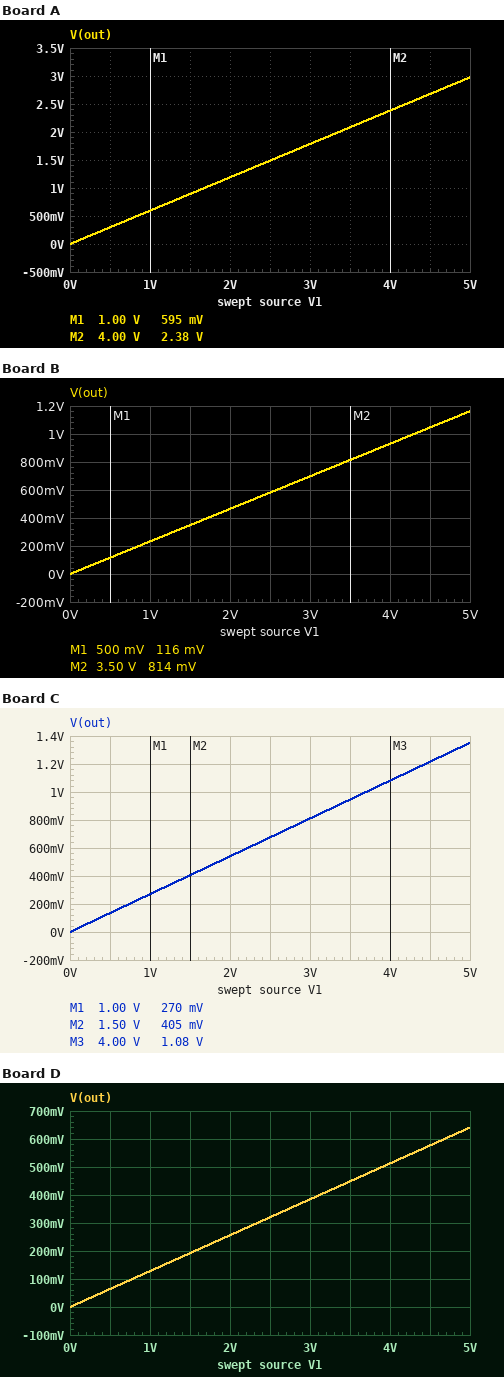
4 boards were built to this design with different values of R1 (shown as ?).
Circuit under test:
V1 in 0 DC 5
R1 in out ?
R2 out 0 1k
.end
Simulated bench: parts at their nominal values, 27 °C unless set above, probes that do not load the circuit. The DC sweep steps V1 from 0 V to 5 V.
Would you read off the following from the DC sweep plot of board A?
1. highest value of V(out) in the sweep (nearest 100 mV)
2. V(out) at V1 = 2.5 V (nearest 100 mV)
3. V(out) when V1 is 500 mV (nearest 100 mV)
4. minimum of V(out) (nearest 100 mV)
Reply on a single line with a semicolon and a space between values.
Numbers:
3.0 V; 1.5 V; 300 mV; 0 V
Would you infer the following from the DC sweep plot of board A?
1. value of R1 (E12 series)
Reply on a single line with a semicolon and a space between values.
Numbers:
680 Ω
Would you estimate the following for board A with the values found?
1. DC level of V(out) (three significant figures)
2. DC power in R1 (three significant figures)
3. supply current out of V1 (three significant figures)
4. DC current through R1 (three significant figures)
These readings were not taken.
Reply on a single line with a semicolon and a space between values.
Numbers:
2.98 V; 6.02 mW; 2.98 mA; 2.98 mA
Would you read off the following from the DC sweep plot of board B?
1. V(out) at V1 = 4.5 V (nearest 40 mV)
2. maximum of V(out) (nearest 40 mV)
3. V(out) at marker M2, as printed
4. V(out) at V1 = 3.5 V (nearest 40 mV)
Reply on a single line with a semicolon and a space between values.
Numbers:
1.04 V; 1.16 V; 814 mV; 800 mV
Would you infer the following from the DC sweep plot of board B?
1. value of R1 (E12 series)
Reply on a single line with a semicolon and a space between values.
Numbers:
3.3 kΩ
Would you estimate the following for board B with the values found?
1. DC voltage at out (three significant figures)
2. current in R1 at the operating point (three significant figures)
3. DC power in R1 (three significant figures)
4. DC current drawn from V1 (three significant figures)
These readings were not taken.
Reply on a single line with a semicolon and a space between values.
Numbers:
1.16 V; 1.16 mA; 4.46 mW; 1.16 mA
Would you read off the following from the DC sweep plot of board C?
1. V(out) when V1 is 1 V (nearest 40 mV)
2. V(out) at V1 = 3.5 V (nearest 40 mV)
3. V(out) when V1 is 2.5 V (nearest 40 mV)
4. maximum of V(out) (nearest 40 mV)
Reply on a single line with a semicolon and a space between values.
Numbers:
280 mV; 960 mV; 680 mV; 1.36 V
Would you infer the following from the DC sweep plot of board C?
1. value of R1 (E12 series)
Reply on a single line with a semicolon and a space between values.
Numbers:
2.7 kΩ
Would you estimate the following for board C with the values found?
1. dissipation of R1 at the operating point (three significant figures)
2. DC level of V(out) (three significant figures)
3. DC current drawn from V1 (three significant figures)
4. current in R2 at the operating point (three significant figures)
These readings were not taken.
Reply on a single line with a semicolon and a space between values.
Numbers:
4.93 mW; 1.35 V; 1.35 mA; 1.35 mA
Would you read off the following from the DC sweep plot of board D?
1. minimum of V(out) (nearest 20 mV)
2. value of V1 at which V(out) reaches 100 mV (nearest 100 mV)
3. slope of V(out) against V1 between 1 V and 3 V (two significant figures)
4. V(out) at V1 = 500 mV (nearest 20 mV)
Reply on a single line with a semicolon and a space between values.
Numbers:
0 V; 800 mV; 0.13 V/V; 60 mV
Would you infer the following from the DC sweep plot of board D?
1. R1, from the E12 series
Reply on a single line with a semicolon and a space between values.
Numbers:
6.8 kΩ
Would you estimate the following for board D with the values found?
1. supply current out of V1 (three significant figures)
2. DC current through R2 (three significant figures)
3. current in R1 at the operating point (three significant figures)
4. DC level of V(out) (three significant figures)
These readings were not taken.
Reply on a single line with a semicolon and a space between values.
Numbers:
641 µA; 641 µA; 641 µA; 641 mV
